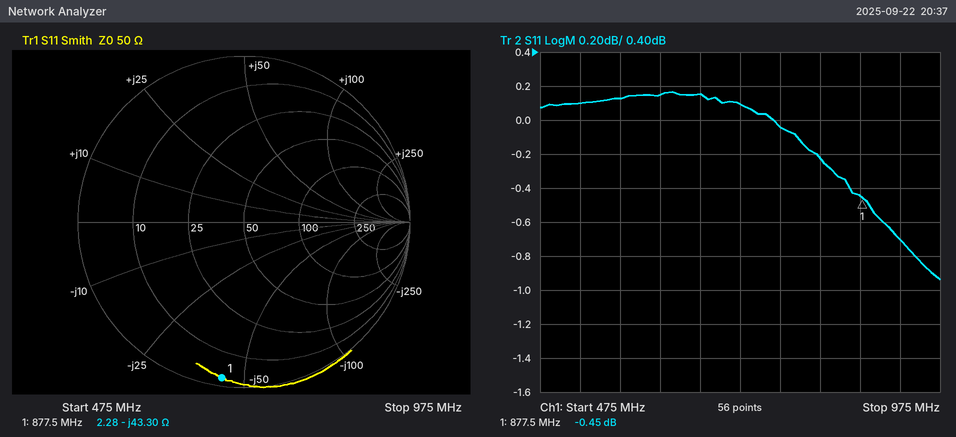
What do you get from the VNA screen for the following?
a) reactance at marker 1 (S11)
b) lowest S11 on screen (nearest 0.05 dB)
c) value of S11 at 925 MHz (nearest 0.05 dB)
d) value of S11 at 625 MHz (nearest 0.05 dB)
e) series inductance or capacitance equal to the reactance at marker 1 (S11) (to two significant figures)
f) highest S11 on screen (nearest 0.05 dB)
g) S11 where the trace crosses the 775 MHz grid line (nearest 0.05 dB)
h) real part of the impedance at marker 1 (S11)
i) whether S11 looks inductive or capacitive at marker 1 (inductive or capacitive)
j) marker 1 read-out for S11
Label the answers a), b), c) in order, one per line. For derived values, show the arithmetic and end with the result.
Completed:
a) -43.30 Ω
b) -0.95 dB
c) -0.70 dB
d) 0.15 dB
e) C = 1/(2π × 877.5 MHz × 43.3 Ω) ≈ 4.2 pF
f) 0.15 dB
g) -0.05 dB
h) 2.28 Ω
i) capacitive
j) -0.45 dB
